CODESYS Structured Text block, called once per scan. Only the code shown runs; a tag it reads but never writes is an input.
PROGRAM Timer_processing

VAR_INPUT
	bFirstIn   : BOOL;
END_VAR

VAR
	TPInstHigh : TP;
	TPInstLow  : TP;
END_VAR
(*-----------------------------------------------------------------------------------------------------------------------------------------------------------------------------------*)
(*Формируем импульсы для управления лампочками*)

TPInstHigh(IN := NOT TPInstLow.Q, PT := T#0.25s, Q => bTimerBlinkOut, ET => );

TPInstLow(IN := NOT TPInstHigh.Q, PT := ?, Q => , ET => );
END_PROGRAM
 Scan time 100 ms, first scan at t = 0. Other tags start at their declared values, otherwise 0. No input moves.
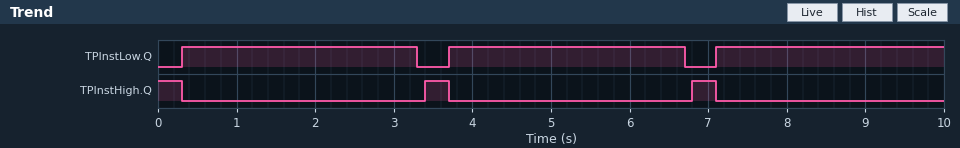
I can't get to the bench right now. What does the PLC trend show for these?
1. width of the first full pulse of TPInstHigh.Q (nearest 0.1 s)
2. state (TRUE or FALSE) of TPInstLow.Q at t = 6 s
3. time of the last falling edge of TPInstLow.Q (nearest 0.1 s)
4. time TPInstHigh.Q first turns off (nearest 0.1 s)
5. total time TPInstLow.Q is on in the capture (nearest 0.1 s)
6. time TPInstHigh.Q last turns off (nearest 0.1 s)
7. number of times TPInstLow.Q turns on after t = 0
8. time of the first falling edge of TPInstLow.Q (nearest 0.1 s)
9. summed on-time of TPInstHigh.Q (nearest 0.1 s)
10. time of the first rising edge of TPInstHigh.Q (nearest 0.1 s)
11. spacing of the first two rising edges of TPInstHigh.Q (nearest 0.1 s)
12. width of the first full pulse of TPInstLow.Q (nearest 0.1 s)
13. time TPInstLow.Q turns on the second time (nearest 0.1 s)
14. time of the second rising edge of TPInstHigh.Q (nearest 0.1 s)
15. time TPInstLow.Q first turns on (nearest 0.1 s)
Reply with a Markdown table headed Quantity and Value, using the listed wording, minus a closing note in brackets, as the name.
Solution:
| Quantity | Value |
|---|---|
| width of the first full pulse of TPInstHigh.Q | 0.3 s |
| state (TRUE or FALSE) of TPInstLow.Q at t = 6 s | TRUE |
| time of the last falling edge of TPInstLow.Q | 6.7 s |
| time TPInstHigh.Q first turns off | 0.3 s |
| total time TPInstLow.Q is on in the capture | 8.9 s |
| time TPInstHigh.Q last turns off | 7.1 s |
| number of times TPInstLow.Q turns on after t = 0 | 3 |
| time of the first falling edge of TPInstLow.Q | 3.3 s |
| summed on-time of TPInstHigh.Q | 0.9 s |
| time of the first rising edge of TPInstHigh.Q | 3.4 s |
| spacing of the first two rising edges of TPInstHigh.Q | 3.4 s |
| width of the first full pulse of TPInstLow.Q | 3.0 s |
| time TPInstLow.Q turns on the second time | 3.7 s |
| time of the second rising edge of TPInstHigh.Q | 6.8 s |
| time TPInstLow.Q first turns on | 0.3 s |
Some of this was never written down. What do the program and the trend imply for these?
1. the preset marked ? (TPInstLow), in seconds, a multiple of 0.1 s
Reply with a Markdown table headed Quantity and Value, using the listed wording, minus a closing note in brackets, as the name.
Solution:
| Quantity | Value |
|---|---|
| the preset marked ? (TPInstLow), in seconds, a multiple of 0.1 s | 3.0 s |
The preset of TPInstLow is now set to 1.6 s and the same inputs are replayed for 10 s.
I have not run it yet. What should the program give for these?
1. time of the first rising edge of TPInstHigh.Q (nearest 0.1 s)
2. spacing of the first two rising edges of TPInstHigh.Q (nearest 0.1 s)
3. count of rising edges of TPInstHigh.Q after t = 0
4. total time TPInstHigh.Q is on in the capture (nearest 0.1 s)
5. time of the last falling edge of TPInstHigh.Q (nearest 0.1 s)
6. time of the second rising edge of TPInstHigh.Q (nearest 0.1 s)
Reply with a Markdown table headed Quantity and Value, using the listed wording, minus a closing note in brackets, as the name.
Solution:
| Quantity | Value |
|---|---|
| time of the first rising edge of TPInstHigh.Q | 2.0 s |
| spacing of the first two rising edges of TPInstHigh.Q | 2.0 s |
| count of rising edges of TPInstHigh.Q after t = 0 | 4 |
| total time TPInstHigh.Q is on in the capture | 1.5 s |
| time of the last falling edge of TPInstHigh.Q | 8.3 s |
| time of the second rising edge of TPInstHigh.Q | 4.0 s |
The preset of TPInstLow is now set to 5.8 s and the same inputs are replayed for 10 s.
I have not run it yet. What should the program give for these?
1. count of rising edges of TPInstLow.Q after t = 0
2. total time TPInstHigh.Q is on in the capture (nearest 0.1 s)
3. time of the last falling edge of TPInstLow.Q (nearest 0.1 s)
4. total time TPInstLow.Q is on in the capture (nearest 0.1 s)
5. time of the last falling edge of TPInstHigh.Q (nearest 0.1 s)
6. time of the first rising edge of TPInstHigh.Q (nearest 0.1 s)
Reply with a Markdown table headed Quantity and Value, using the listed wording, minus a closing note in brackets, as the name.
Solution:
| Quantity | Value |
|---|---|
| count of rising edges of TPInstLow.Q after t = 0 | 2 |
| total time TPInstHigh.Q is on in the capture | 0.6 s |
| time of the last falling edge of TPInstLow.Q | 6.1 s |
| total time TPInstLow.Q is on in the capture | 9.3 s |
| time of the last falling edge of TPInstHigh.Q | 6.5 s |
| time of the first rising edge of TPInstHigh.Q | 6.2 s |
